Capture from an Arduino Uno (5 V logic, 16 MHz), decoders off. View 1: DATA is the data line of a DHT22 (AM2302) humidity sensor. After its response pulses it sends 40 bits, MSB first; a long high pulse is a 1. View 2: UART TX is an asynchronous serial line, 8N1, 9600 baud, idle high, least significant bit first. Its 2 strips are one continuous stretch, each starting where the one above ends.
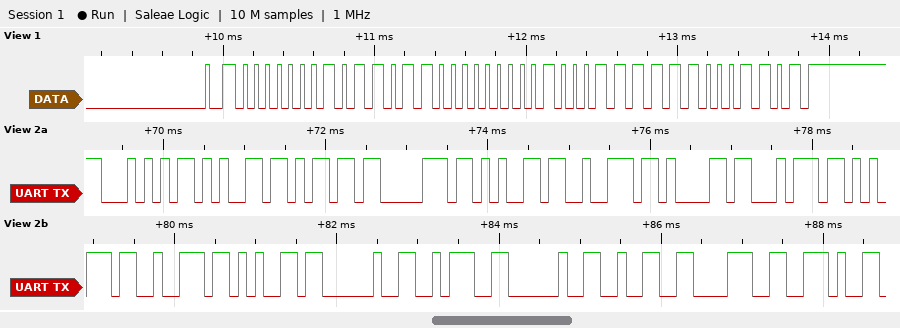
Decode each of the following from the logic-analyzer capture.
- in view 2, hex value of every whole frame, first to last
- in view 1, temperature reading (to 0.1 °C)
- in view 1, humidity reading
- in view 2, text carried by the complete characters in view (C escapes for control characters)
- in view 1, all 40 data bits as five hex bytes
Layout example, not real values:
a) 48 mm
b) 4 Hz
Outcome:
a) 0x54 0x65 0x6D 0x70 0x65 0x72 0x61 0x74 0x75 0x72 0x65 0x20 0x3A 0x20 0x32 0x38 0x2E
b) 28.7 °C
c) 36.4 %
d) "Temperature : 28."
e) 01 6C 01 1F 8D
